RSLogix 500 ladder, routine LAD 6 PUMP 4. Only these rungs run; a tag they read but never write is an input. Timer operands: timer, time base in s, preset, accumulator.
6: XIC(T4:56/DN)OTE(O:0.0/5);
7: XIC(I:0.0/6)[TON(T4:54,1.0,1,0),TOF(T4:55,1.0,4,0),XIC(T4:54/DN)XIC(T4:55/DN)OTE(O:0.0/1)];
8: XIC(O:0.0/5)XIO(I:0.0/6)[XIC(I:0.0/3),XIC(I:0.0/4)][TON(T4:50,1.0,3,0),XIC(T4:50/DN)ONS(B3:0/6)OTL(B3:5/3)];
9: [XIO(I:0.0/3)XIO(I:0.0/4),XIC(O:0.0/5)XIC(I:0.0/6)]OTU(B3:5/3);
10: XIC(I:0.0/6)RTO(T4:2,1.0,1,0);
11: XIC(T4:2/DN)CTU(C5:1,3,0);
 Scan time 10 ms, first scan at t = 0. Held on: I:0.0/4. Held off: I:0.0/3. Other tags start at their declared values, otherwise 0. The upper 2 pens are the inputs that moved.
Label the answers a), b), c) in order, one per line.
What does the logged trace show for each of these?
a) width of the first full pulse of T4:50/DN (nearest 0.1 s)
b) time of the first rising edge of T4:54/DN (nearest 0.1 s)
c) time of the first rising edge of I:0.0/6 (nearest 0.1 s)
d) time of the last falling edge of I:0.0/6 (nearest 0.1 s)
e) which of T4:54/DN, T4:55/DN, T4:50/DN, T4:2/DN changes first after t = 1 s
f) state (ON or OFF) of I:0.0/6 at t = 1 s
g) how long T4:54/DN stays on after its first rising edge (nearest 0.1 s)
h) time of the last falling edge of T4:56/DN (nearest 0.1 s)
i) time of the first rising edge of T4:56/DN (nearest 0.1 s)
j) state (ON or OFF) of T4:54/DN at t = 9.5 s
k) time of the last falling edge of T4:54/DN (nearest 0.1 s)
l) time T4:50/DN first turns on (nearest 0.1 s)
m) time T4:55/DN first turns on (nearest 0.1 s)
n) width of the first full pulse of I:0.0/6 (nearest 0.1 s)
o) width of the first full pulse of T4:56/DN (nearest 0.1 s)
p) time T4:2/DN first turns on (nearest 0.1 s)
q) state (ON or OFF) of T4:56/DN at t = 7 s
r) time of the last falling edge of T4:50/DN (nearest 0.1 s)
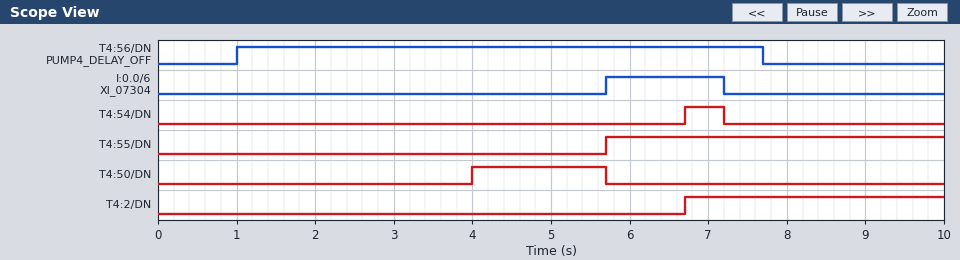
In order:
a) 1.7 s
b) 6.7 s
c) 5.7 s
d) 7.2 s
e) T4:50/DN
f) OFF
g) 0.5 s
h) 7.7 s
i) 1.0 s
j) OFF
k) 7.2 s
l) 4.0 s
m) 5.7 s
n) 1.5 s
o) 6.7 s
p) 6.7 s
q) ON
r) 5.7 s
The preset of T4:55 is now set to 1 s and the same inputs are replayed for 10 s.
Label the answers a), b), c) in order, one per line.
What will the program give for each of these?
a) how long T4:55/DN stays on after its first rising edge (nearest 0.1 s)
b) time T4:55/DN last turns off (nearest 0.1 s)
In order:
a) 2.5 s
b) 8.2 s
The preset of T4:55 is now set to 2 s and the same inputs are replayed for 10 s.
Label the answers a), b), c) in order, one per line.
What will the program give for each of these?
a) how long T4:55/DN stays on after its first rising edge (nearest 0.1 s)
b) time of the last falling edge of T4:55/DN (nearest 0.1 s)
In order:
a) 3.5 s
b) 9.2 s
